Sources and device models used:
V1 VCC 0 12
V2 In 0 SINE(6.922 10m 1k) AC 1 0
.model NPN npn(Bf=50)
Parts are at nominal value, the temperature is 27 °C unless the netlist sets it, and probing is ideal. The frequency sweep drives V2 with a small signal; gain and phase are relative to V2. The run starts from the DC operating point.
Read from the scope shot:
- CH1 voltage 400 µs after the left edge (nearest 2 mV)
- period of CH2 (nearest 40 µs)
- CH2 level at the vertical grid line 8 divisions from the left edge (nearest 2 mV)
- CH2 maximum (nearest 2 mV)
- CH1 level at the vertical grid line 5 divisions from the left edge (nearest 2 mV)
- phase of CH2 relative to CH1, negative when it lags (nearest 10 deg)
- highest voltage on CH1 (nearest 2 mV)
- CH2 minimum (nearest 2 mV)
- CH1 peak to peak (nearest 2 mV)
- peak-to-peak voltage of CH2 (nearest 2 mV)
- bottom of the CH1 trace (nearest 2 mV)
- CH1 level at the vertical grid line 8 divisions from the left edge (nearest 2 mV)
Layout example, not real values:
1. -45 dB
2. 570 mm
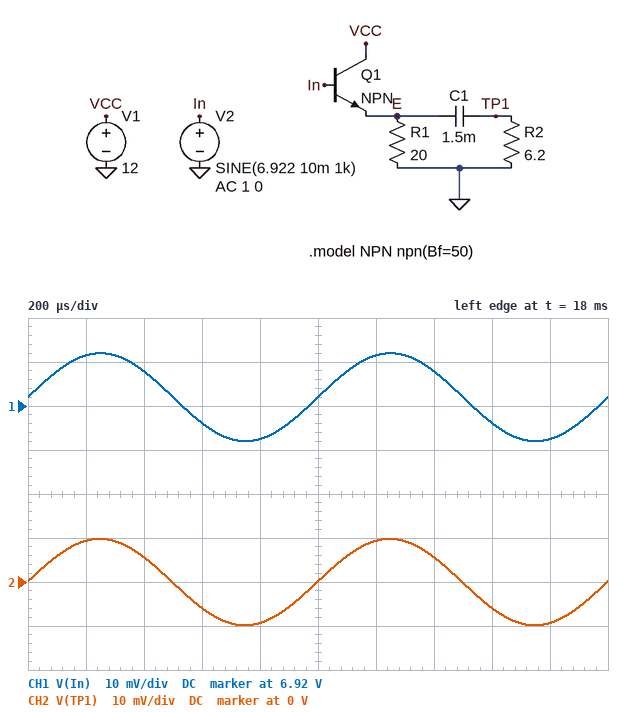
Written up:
1. 6.928 V
2. 1.00 ms
3. -6 mV
4. 10 mV
5. 6.922 V
6. 0 deg
7. 6.932 V
8. -10 mV
9. 20 mV
10. 20 mV
11. 6.912 V
12. 6.916 V
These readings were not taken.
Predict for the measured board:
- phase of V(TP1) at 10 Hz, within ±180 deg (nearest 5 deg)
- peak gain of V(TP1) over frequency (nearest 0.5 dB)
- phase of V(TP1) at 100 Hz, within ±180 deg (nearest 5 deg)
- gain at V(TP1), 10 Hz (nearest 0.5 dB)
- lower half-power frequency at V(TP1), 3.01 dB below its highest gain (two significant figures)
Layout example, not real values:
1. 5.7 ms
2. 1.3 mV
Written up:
1. 60 deg
2. 0 dB
3. 10 deg
4. -6.0 dB
5. 17 Hz
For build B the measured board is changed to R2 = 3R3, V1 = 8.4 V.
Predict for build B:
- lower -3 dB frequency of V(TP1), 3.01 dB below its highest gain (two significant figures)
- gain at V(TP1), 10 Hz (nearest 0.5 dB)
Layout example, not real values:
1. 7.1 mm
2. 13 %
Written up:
1. 31 Hz
2. -10.5 dB
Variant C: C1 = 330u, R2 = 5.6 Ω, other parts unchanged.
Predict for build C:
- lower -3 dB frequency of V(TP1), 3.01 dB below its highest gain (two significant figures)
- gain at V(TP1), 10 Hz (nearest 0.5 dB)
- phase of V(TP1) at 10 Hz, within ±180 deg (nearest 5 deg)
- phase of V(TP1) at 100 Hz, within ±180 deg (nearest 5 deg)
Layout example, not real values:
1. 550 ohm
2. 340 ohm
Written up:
1. 85 Hz
2. -19.0 dB
3. 85 deg
4. 40 deg
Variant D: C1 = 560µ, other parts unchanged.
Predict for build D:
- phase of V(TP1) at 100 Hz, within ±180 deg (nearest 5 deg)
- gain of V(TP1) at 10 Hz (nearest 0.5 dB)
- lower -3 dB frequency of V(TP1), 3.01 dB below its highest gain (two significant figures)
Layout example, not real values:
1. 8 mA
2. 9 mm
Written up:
1. 25 deg
2. -13.5 dB
3. 45 Hz
